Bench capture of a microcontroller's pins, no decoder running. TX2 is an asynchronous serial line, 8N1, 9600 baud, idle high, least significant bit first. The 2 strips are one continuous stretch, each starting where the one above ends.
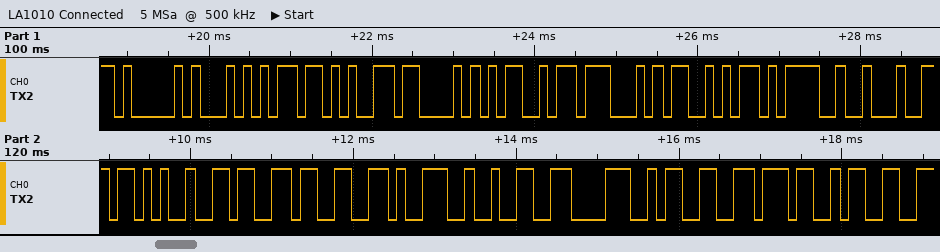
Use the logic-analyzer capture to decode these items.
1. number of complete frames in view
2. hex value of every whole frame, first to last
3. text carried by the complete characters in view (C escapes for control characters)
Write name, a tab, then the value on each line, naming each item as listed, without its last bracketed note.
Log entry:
number of complete frames in view	18
hex value of every whole frame, first to last	41 54 2B 43 4D 47 53 3D 22 2B 36 33 39 32 38 33 37 33
text carried by the complete characters in view	"AT+CMGS=\"+63928373"
